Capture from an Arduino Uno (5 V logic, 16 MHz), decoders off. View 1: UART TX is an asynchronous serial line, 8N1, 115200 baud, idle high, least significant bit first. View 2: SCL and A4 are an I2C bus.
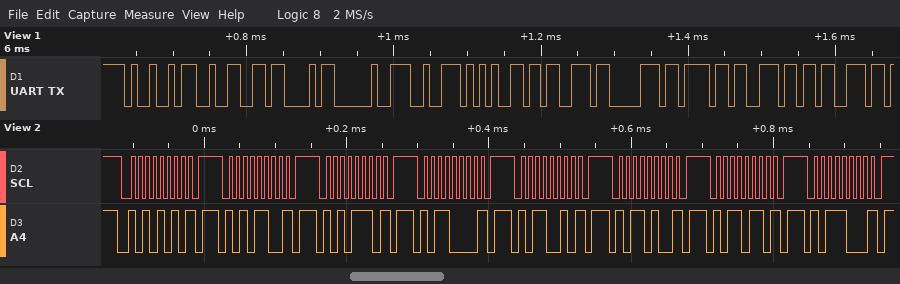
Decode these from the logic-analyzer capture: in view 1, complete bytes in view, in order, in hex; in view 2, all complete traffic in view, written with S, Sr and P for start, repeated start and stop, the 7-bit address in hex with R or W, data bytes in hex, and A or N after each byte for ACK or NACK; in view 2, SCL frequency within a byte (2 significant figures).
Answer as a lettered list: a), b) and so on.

a) 49 32 43 20 72 65 73 70 6F 6E 73
b) S 55W N P S 56W N P S 57W N P S 58W N P S 59W N P S 5AW N P S 5BW N P S 5CW N P
c) 100 kHz
